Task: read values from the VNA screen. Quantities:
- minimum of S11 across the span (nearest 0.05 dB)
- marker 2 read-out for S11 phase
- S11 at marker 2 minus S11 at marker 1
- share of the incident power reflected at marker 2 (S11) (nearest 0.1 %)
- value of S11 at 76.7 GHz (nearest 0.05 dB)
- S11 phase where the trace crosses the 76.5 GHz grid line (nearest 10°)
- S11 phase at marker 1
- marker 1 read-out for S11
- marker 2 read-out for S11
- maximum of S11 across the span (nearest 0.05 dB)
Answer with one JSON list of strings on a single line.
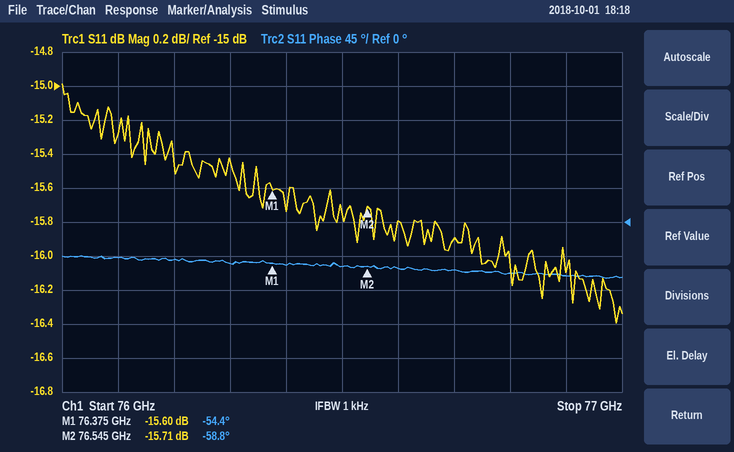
["-16.40 dB", "-58.8°", "-0.11 dB", "2.7 %", "-15.90 dB", "-60°", "-54.4°", "-15.60 dB", "-15.71 dB", "-15.00 dB"]
